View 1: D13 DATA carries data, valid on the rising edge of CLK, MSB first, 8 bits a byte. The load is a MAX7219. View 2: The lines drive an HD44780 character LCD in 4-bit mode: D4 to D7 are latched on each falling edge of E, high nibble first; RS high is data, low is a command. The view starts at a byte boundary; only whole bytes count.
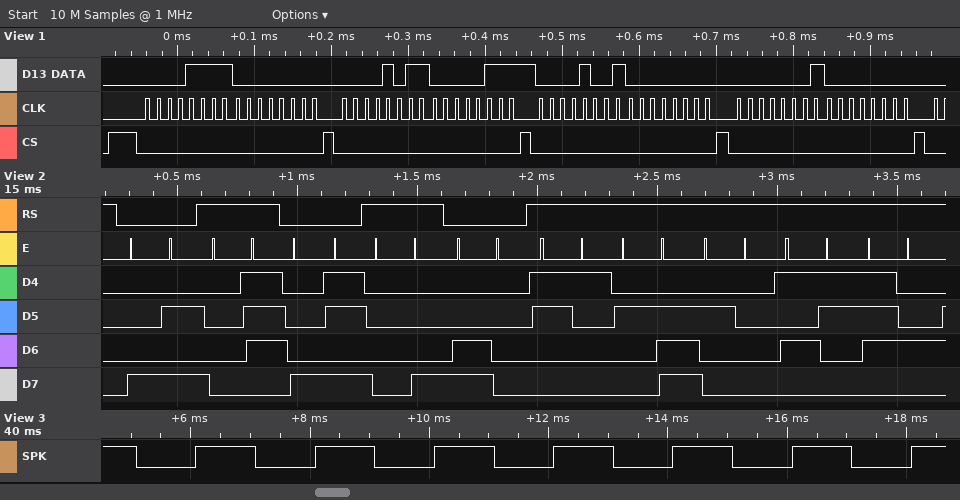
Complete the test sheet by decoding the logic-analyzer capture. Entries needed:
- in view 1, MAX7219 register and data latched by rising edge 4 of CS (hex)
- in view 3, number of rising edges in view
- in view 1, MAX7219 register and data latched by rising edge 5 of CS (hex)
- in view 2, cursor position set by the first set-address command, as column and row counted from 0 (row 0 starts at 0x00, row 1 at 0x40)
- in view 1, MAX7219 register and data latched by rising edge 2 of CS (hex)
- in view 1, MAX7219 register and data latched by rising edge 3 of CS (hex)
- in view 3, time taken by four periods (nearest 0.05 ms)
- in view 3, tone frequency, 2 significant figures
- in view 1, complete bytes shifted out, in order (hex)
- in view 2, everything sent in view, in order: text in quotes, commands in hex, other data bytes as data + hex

register 0x9, data 0x00
7
register 0x1, data 0x00
column 10, row 0
register 0xF, data 0x00
register 0xB, data 0x07
8.00 ms
500 Hz
0x0F 0x00 0x0B 0x07 0x09 0x00 0x01 0x00
0x8A data 07 0x8B data 08 0xC0 "1. St"
